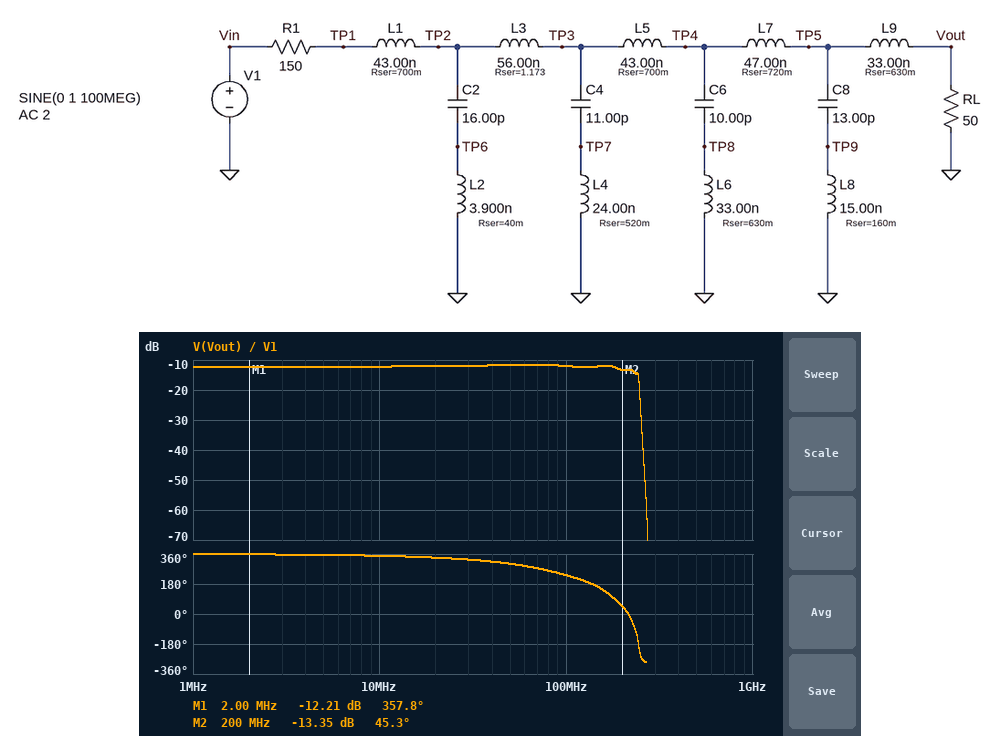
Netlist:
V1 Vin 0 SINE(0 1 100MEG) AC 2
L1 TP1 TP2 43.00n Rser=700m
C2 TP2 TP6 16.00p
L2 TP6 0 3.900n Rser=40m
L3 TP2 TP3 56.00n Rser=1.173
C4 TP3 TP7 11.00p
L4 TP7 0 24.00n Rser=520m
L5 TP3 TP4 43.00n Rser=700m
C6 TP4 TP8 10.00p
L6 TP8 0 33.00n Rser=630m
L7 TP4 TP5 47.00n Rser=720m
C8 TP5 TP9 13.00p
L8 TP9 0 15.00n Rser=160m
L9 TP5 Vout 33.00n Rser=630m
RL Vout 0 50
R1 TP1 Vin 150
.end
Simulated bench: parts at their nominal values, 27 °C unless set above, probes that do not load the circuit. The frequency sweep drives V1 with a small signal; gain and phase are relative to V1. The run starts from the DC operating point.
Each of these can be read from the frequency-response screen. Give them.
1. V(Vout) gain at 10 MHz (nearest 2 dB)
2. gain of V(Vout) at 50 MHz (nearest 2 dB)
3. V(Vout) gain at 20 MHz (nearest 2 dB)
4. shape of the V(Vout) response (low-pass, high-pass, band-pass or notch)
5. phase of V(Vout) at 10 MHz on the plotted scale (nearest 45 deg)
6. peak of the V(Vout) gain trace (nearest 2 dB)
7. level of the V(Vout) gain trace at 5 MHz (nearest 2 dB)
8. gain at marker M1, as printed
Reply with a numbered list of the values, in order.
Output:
1. -12 dB
2. -12 dB
3. -12 dB
4. low-pass
5. 360 deg
6. -12 dB
7. -12 dB
8. -12.21 dB
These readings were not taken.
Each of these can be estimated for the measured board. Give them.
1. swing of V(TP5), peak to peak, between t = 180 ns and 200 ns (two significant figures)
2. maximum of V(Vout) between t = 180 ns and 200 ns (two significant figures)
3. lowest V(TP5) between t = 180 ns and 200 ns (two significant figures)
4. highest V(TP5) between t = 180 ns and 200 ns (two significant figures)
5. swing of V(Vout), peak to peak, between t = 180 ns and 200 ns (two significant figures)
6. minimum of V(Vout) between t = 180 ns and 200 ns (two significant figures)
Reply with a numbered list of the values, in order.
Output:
1. 550 mV
2. 250 mV
3. -270 mV
4. 270 mV
5. 500 mV
6. -250 mV
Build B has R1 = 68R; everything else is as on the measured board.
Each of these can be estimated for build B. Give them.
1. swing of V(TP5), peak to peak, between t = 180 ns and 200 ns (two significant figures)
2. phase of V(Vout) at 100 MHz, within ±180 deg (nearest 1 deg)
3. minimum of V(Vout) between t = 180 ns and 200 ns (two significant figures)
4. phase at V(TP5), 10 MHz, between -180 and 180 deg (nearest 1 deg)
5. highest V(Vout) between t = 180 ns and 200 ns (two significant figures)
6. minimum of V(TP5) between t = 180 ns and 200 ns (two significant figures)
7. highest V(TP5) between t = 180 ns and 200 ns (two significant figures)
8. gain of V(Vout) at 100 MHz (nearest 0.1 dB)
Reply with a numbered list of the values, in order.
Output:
1. 900 mV
2. -127 deg
3. -410 mV
4. -10 deg
5. 410 mV
6. -450 mV
7. 450 mV
8. -7.7 dB
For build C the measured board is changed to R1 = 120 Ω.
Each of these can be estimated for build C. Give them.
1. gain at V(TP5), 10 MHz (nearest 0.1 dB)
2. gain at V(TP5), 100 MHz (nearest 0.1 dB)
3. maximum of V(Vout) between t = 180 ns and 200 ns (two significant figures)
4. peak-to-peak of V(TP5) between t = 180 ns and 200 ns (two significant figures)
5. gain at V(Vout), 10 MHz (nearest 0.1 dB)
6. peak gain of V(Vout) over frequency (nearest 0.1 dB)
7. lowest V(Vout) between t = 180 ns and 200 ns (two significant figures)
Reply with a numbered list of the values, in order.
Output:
1. -10.7 dB
2. -9.9 dB
3. 290 mV
4. 640 mV
5. -10.8 dB
6. -10.3 dB
7. -290 mV
